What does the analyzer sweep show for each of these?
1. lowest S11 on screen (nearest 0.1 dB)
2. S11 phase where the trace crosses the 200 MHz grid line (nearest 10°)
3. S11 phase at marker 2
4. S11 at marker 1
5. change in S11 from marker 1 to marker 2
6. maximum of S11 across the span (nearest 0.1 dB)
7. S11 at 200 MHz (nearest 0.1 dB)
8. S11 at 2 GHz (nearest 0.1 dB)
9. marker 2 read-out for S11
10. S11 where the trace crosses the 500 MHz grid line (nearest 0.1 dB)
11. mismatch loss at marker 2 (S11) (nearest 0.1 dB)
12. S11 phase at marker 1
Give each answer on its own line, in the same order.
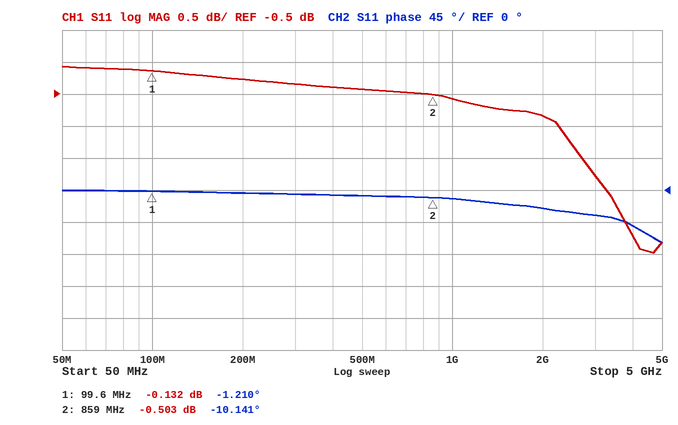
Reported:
-3.0 dB
0°
-10.141°
-0.132 dB
-0.371 dB
-0.1 dB
-0.3 dB
-0.8 dB
-0.503 dB
-0.4 dB
9.6 dB
-1.210°
